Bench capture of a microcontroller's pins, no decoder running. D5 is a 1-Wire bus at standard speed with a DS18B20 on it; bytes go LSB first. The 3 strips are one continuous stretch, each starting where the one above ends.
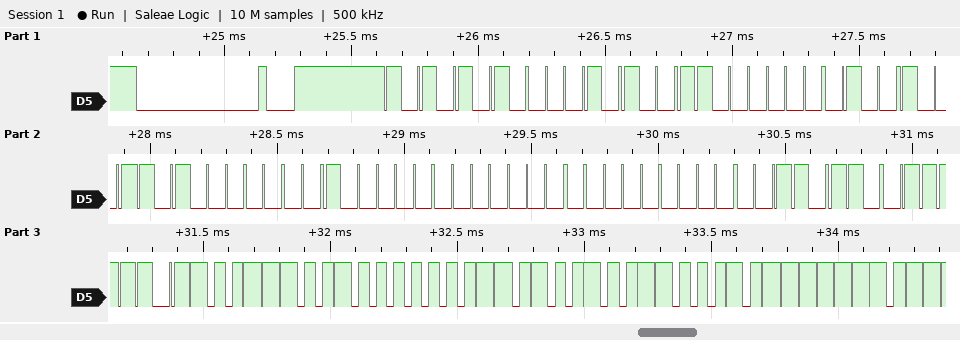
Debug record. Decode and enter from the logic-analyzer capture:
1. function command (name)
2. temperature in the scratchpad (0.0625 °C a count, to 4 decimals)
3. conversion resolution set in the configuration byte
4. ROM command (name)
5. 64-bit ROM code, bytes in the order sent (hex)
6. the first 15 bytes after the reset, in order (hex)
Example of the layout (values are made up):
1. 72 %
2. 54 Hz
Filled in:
1. Read Scratchpad
2. 19.5625 °C
3. 12 bits
4. Match ROM
5. 28 03 92 05 04 00 00 6C
6. 55 28 03 92 05 04 00 00 6C BE 39 01 4B 46 7F
